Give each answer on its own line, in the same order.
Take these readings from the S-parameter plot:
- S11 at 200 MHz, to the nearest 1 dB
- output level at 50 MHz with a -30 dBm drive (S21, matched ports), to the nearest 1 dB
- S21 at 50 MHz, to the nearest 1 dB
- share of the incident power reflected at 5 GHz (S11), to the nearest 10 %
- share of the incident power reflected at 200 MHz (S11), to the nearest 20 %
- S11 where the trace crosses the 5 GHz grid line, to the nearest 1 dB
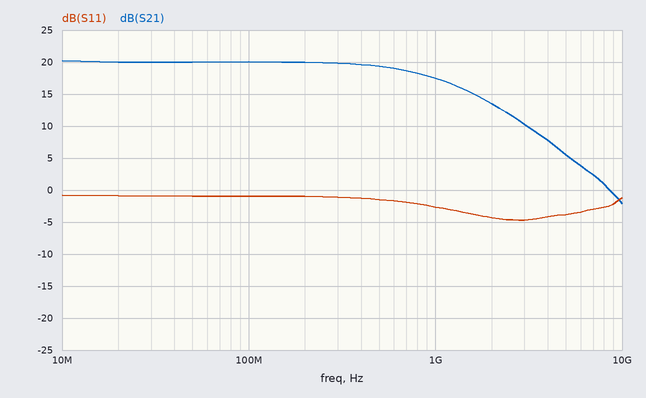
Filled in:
-1 dB
-10 dBm
20 dB
40 %
80 %
-4 dB
